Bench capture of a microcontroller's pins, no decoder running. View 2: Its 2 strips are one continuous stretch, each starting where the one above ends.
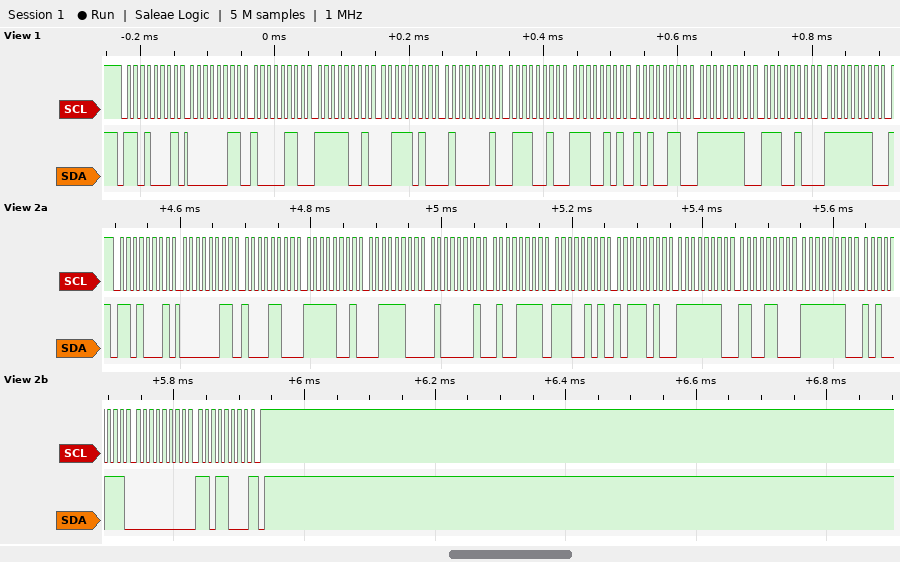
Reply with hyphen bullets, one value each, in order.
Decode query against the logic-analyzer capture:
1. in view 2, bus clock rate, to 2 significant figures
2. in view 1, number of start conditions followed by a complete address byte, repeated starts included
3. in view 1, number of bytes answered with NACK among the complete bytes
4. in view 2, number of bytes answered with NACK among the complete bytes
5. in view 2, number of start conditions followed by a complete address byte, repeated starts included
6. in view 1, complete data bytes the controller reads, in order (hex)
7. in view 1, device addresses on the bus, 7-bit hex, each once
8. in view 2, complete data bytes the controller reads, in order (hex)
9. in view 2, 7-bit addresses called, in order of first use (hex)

- 100 kHz
- 1
- 0
- 1
- 1
- 03 86 F9 3A 41 72 E5 A6 FE E4 FE
- 0x68
- 03 8C F9 3C 41 4F E5 BA FE CC FE A7 00 D8
- 0x68
